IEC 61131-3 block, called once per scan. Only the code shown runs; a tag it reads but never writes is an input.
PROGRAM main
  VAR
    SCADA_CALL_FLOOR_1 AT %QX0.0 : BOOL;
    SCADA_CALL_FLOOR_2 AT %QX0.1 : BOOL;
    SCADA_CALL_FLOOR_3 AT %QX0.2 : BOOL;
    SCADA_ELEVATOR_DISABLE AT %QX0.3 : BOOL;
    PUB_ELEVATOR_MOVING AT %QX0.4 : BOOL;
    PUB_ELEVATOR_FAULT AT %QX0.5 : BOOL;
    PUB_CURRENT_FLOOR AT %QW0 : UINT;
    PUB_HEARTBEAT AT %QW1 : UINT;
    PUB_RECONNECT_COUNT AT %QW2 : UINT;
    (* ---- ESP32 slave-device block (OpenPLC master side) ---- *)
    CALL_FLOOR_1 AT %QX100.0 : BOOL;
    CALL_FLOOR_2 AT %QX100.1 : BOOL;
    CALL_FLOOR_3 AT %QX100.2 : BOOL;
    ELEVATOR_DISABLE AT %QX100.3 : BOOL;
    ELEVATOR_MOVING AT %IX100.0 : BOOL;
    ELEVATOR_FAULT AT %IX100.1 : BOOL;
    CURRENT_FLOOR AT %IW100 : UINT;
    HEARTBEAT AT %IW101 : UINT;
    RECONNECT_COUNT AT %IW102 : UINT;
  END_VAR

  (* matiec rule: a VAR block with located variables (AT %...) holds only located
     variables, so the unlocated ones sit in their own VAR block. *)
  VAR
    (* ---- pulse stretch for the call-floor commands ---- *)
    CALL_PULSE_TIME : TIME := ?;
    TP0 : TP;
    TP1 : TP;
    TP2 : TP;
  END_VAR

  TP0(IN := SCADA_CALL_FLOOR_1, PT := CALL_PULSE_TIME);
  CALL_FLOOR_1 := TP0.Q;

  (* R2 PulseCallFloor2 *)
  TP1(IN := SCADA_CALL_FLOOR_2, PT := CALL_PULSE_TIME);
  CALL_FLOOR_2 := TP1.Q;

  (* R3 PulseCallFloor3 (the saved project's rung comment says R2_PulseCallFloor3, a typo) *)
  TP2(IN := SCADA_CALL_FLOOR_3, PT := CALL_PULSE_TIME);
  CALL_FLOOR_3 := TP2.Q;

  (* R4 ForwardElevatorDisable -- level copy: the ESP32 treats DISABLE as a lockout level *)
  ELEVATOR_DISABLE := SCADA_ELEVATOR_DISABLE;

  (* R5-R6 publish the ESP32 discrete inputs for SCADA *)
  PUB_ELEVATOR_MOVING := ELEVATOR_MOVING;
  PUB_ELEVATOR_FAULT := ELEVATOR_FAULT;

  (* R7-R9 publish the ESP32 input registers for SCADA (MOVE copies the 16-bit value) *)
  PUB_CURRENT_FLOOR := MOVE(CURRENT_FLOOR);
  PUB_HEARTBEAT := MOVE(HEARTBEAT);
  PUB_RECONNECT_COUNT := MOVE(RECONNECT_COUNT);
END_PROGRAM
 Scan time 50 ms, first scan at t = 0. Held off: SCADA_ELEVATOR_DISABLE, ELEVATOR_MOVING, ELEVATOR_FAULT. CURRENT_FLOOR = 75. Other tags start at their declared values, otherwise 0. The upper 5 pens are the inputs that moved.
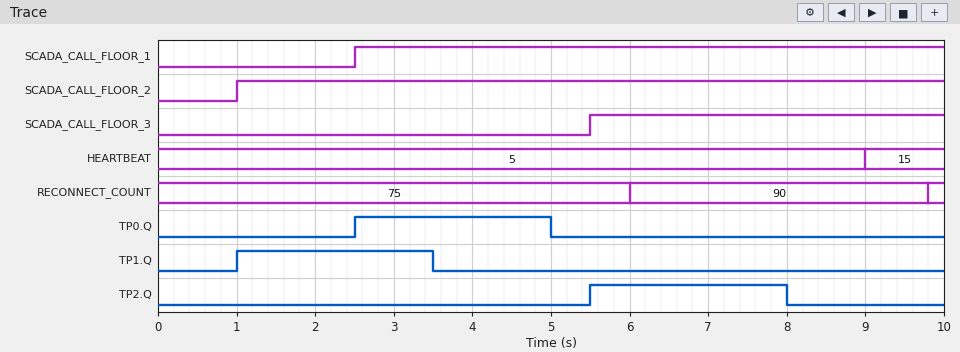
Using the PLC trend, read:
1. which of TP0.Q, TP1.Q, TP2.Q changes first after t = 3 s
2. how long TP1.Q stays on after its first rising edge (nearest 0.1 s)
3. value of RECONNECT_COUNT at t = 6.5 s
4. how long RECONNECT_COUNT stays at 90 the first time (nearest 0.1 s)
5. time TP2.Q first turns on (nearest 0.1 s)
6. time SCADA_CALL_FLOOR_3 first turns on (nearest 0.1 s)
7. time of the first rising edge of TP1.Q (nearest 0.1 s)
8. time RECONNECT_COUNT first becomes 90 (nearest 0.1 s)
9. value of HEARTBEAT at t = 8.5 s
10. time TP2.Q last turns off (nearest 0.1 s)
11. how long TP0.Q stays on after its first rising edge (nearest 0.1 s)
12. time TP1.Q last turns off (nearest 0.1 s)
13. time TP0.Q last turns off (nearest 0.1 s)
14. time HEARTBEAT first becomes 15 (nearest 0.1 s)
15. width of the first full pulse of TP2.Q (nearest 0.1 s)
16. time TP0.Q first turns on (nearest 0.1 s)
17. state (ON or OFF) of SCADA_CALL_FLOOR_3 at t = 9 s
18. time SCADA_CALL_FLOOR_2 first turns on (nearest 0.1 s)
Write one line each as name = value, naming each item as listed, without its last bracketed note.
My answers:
which of TP0.Q, TP1.Q, TP2.Q changes first after t = 3 s = TP1.Q
how long TP1.Q stays on after its first rising edge = 2.5 s
value of RECONNECT_COUNT at t = 6.5 s = 90
how long RECONNECT_COUNT stays at 90 the first time = 3.8 s
time TP2.Q first turns on = 5.5 s
time SCADA_CALL_FLOOR_3 first turns on = 5.5 s
time of the first rising edge of TP1.Q = 1.0 s
time RECONNECT_COUNT first becomes 90 = 6.0 s
value of HEARTBEAT at t = 8.5 s = 5
time TP2.Q last turns off = 8.0 s
how long TP0.Q stays on after its first rising edge = 2.5 s
time TP1.Q last turns off = 3.5 s
time TP0.Q last turns off = 5.0 s
time HEARTBEAT first becomes 15 = 9.0 s
width of the first full pulse of TP2.Q = 2.5 s
time TP0.Q first turns on = 2.5 s
state (ON or OFF) of SCADA_CALL_FLOOR_3 at t = 9 s = ON
time SCADA_CALL_FLOOR_2 first turns on = 1.0 s
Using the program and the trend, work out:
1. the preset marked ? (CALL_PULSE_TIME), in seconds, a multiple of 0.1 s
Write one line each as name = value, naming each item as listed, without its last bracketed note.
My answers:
the preset marked ? (CALL_PULSE_TIME), in seconds, a multiple of 0.1 s = 2.5 s
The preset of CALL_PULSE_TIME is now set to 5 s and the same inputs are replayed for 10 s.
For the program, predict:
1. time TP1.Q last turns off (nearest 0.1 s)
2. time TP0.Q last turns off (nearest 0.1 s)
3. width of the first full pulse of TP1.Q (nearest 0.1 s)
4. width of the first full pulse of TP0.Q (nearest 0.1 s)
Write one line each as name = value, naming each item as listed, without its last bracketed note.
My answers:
time TP1.Q last turns off = 6.0 s
time TP0.Q last turns off = 7.5 s
width of the first full pulse of TP1.Q = 5.0 s
width of the first full pulse of TP0.Q = 5.0 s
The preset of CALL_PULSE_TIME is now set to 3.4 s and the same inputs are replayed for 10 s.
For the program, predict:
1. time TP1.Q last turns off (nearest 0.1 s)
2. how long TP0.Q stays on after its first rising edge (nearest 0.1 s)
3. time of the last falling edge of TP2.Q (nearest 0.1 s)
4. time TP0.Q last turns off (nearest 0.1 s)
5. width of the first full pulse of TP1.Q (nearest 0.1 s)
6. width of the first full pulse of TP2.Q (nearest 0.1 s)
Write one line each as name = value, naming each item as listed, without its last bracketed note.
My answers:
time TP1.Q last turns off = 4.4 s
how long TP0.Q stays on after its first rising edge = 3.4 s
time of the last falling edge of TP2.Q = 8.9 s
time TP0.Q last turns off = 5.9 s
width of the first full pulse of TP1.Q = 3.4 s
width of the first full pulse of TP2.Q = 3.4 s
